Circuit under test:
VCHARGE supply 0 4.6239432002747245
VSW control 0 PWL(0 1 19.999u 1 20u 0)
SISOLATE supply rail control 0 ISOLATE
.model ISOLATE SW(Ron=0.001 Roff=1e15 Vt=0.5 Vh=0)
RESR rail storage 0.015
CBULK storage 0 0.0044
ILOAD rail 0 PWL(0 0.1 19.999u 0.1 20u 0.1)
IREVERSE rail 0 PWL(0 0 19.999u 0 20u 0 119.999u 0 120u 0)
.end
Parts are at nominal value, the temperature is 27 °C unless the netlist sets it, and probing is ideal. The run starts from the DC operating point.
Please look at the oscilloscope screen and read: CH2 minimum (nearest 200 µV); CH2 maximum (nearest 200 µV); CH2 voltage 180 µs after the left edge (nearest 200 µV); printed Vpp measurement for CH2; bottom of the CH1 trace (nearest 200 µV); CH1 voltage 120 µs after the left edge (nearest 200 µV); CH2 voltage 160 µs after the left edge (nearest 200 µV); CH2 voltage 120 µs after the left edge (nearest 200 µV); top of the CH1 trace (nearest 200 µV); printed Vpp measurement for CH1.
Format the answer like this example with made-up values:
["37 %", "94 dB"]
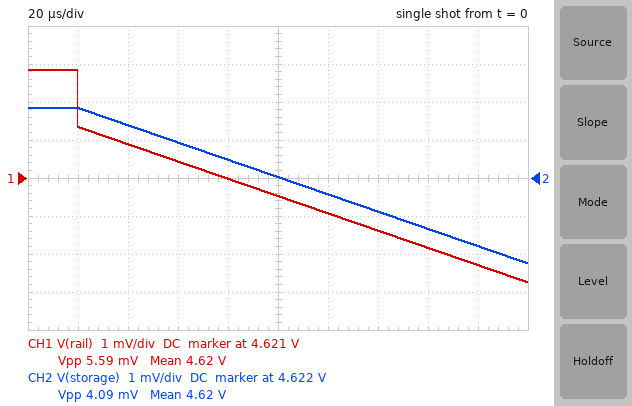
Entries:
["4.6198 V", "4.6238 V", "4.6202 V", "4.09 mV", "4.6182 V", "4.6200 V", "4.6206 V", "4.6216 V", "4.6238 V", "5.59 mV"]
